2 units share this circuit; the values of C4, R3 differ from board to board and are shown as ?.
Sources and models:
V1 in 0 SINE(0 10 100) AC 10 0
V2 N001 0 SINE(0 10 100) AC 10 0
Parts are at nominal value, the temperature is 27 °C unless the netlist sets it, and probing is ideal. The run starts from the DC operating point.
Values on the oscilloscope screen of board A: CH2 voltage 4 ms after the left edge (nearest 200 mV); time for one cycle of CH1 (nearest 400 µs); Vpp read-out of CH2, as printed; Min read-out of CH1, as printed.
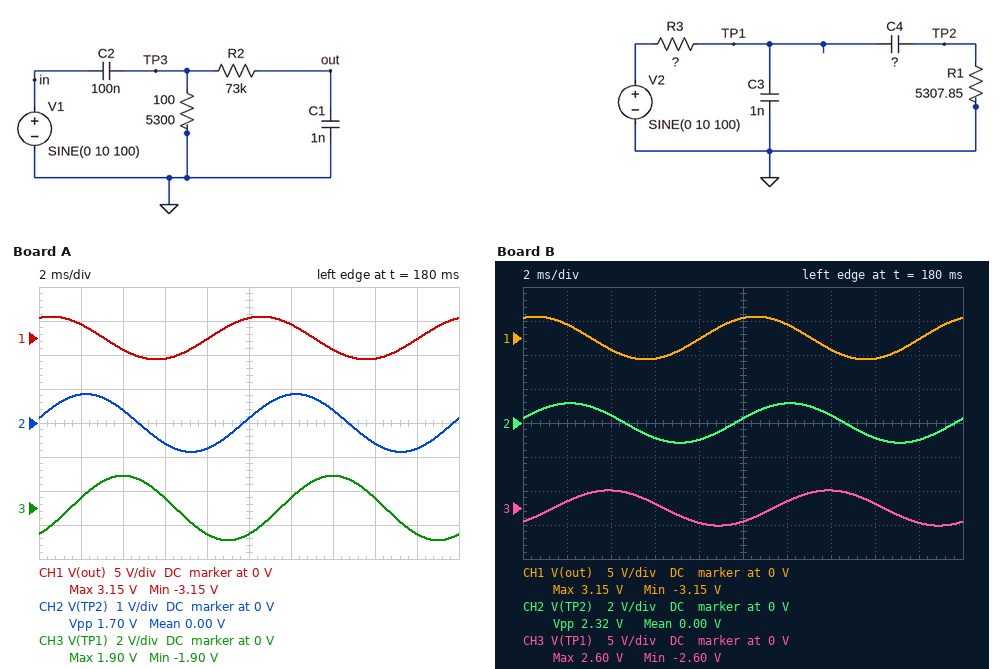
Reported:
400 mV
10.0 ms
1.70 V
-3.15 V
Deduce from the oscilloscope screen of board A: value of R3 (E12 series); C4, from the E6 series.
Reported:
56 kΩ
150 nF
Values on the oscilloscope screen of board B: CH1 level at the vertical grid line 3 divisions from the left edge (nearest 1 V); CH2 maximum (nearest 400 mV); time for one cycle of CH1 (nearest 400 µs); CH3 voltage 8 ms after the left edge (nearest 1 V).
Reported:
-3 V
1.2 V
10.0 ms
-2 V
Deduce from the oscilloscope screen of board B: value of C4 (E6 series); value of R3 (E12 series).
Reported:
150 nF
39 kΩ
